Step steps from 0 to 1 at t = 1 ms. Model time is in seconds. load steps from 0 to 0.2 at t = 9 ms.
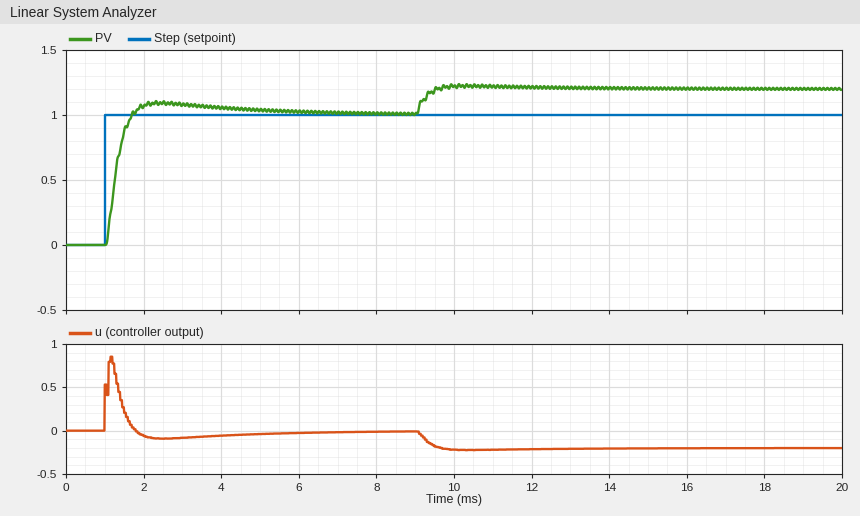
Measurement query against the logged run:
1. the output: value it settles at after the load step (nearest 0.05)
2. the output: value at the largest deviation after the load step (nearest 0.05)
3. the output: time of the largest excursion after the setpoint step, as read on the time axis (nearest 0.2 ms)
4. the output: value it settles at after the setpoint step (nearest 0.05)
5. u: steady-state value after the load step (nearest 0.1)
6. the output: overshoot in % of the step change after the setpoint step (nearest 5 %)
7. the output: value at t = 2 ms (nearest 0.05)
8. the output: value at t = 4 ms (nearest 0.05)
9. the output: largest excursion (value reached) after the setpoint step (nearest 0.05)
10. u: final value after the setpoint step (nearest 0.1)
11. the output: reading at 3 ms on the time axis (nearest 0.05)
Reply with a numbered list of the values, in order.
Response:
1. 1.20
2. 1.25
3. 2.4 ms
4. 1.00
5. -0.2
6. 10 %
7. 1.05
8. 1.05
9. 1.10
10. 0.0
11. 1.10
